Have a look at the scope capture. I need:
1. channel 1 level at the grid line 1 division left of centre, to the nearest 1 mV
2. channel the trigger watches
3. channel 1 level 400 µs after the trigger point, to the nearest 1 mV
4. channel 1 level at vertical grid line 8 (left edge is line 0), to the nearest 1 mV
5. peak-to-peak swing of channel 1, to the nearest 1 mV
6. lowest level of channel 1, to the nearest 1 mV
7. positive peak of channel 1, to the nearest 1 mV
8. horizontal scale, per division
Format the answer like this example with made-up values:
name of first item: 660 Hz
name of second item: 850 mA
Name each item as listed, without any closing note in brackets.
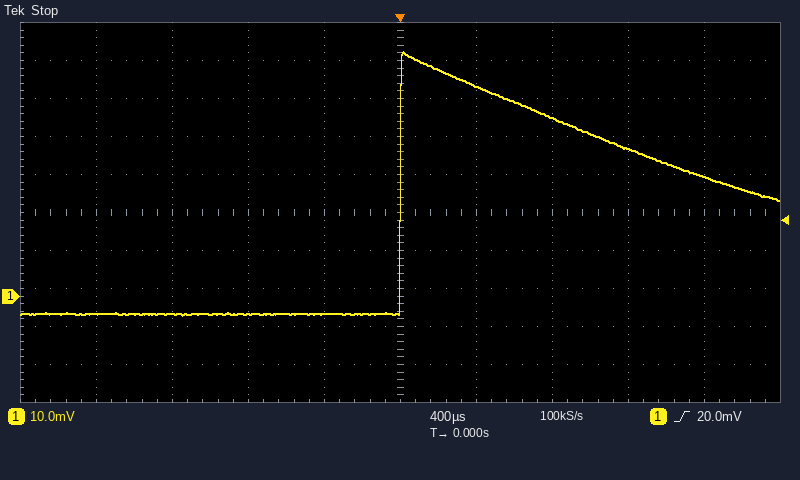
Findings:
channel 1 level at the grid line 1 division left of centre, to the nearest 1 mV: -5 mV
channel the trigger watches: channel 1
channel 1 level 400 µs after the trigger point, to the nearest 1 mV: 55 mV
channel 1 level at vertical grid line 8 (left edge is line 0), to the nearest 1 mV: 39 mV
peak-to-peak swing of channel 1, to the nearest 1 mV: 69 mV
lowest level of channel 1, to the nearest 1 mV: -5 mV
positive peak of channel 1, to the nearest 1 mV: 64 mV
horizontal scale, per division: 400 µs
